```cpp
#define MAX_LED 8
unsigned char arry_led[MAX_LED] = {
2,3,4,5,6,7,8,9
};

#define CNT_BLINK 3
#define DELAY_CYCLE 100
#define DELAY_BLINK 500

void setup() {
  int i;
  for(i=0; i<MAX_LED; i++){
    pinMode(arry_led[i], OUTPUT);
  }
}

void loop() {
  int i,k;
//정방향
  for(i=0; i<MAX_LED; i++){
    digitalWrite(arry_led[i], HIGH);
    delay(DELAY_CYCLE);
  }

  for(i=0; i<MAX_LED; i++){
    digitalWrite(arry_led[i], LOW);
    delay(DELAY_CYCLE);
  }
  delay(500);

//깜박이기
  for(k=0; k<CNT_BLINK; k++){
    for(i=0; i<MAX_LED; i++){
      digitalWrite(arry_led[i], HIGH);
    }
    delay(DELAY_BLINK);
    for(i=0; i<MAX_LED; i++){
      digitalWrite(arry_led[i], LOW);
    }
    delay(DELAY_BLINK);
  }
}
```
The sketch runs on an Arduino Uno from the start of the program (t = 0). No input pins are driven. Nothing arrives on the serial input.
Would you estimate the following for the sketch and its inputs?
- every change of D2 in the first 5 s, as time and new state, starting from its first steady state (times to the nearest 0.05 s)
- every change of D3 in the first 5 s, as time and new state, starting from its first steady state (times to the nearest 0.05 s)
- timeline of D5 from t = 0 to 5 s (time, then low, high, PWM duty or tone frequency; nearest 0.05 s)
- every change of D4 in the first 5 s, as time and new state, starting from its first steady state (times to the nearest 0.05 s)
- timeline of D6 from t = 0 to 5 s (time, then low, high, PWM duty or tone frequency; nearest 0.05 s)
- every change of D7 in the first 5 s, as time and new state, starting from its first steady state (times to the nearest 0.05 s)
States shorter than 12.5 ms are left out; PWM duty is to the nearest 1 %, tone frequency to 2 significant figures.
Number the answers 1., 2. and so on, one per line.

1. 0 s high; 0.8 s low; 2.1 s high; 2.6 s low; 3.1 s high; 3.6 s low; 4.1 s high; 4.6 s low
2. 0 s low; 0.1 s high; 0.9 s low; 2.1 s high; 2.6 s low; 3.1 s high; 3.6 s low; 4.1 s high; 4.6 s low
3. 0 s low; 0.3 s high; 1.1 s low; 2.1 s high; 2.6 s low; 3.1 s high; 3.6 s low; 4.1 s high; 4.6 s low
4. 0 s low; 0.2 s high; 1 s low; 2.1 s high; 2.6 s low; 3.1 s high; 3.6 s low; 4.1 s high; 4.6 s low
5. 0 s low; 0.4 s high; 1.2 s low; 2.1 s high; 2.6 s low; 3.1 s high; 3.6 s low; 4.1 s high; 4.6 s low
6. 0 s low; 0.5 s high; 1.3 s low; 2.1 s high; 2.6 s low; 3.1 s high; 3.6 s low; 4.1 s high; 4.6 s low
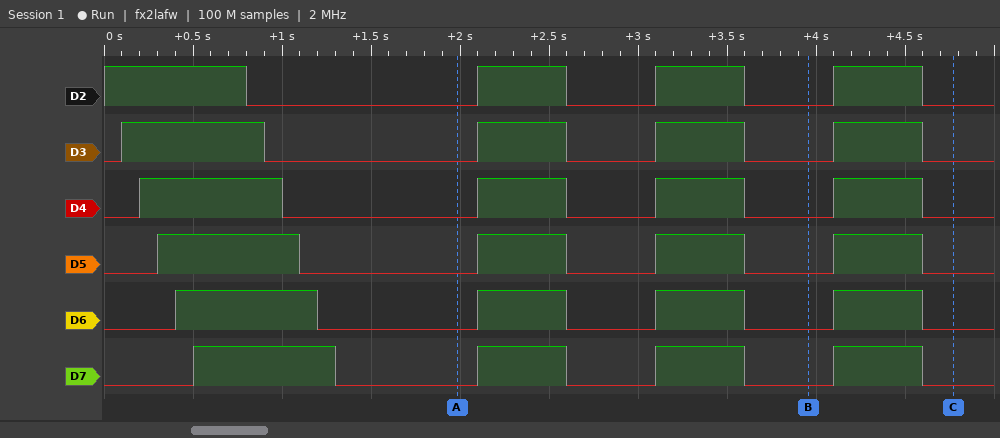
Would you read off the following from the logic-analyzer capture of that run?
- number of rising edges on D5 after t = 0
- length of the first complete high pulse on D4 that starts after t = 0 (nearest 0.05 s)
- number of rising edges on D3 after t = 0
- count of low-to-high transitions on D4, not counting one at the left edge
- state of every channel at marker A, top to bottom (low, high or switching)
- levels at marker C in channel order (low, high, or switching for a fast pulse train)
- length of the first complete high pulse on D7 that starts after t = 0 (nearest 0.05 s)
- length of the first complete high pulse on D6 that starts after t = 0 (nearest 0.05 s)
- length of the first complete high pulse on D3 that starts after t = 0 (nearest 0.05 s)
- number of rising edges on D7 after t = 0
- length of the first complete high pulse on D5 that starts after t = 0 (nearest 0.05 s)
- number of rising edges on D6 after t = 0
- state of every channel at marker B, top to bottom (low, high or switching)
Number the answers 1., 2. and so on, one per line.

1. 4
2. 0.80 s
3. 4
4. 4
5. D2 low, D3 low, D4 low, D5 low, D6 low, D7 low
6. D2 low, D3 low, D4 low, D5 low, D6 low, D7 low
7. 0.80 s
8. 0.80 s
9. 0.80 s
10. 4
11. 0.80 s
12. 4
13. D2 low, D3 low, D4 low, D5 low, D6 low, D7 low
